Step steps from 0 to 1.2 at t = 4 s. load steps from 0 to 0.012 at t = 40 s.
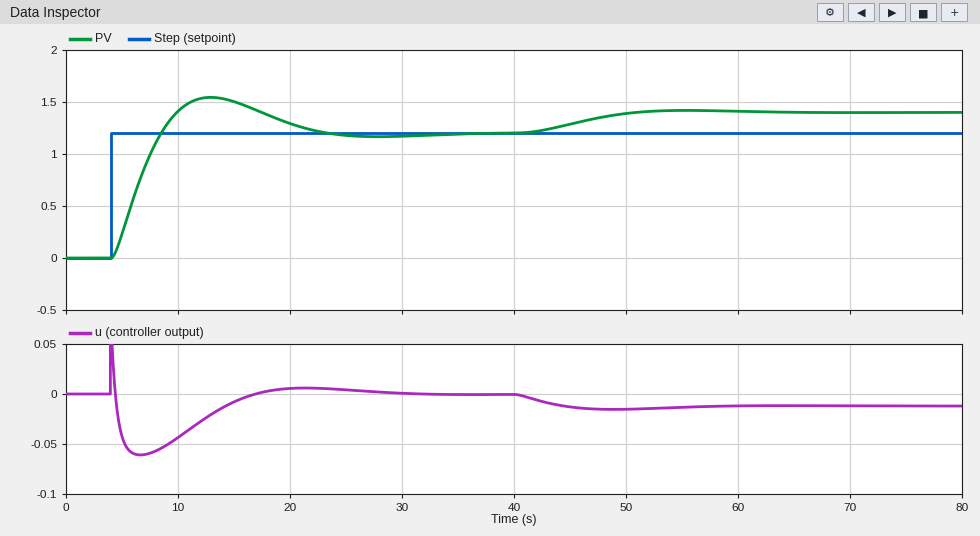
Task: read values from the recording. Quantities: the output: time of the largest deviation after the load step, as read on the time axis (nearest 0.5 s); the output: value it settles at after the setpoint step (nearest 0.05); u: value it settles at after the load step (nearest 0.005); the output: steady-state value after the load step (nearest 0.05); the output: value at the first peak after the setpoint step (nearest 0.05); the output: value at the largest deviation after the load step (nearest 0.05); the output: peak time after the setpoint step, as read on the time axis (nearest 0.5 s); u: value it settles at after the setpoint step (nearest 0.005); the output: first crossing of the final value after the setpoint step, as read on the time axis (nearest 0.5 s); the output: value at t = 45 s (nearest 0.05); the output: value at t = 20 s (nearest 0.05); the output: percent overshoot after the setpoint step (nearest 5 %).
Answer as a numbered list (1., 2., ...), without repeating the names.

1. 55.5 s
2. 1.20
3. -0.010
4. 1.40
5. 1.55
6. 1.40
7. 13.0 s
8. 0.000
9. 8.5 s
10. 1.30
11. 1.30
12. 30 %
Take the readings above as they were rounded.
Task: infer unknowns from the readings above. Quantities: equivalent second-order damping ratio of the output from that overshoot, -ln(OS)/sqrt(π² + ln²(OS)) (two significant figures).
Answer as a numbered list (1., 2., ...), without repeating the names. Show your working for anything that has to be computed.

1. ln(0.3) = -1.204; 1.204 / sqrt(9.870 + 1.450) = 0.36
